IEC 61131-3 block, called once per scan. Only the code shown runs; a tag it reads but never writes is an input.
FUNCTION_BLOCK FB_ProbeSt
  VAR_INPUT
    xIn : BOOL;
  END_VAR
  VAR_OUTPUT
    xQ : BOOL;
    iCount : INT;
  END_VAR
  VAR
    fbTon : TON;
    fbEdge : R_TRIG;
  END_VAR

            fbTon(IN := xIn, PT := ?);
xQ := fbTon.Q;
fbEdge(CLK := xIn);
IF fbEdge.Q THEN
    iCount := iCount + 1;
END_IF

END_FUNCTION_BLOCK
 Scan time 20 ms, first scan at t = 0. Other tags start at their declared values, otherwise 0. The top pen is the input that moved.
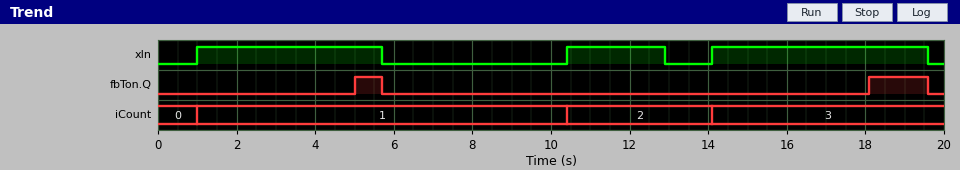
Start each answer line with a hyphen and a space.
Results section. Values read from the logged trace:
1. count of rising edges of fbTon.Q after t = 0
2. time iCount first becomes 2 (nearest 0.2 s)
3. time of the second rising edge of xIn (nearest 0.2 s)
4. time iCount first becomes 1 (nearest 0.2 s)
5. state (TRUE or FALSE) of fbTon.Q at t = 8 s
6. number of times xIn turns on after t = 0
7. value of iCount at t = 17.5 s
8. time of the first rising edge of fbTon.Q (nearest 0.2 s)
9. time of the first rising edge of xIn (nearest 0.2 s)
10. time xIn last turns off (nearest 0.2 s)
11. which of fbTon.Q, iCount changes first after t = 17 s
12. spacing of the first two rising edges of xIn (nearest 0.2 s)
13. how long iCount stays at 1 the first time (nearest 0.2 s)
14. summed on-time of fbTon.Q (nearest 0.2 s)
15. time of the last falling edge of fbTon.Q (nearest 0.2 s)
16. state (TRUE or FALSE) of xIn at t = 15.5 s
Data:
- 2
- 10.4 s
- 10.4 s
- 1.0 s
- FALSE
- 3
- 3
- 5.0 s
- 1.0 s
- 19.6 s
- fbTon.Q
- 9.4 s
- 9.4 s
- 2.2 s
- 19.6 s
- TRUE
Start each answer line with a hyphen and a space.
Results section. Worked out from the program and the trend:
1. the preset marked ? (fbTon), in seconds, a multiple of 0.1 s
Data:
- 4.0 s
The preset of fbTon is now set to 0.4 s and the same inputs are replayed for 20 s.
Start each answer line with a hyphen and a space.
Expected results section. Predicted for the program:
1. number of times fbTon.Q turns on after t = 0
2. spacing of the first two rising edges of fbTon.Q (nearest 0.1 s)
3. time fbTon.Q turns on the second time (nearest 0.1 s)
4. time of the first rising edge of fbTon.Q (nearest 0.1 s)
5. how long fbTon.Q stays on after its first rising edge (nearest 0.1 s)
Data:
- 3
- 9.4 s
- 10.8 s
- 1.4 s
- 4.3 s
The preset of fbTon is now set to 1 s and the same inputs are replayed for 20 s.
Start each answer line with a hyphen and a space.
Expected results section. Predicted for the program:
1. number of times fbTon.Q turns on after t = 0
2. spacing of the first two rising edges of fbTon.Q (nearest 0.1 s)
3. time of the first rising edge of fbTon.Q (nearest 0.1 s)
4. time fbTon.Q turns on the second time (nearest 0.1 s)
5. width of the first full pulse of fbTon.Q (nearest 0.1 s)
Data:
- 3
- 9.4 s
- 2.0 s
- 11.4 s
- 3.7 s
